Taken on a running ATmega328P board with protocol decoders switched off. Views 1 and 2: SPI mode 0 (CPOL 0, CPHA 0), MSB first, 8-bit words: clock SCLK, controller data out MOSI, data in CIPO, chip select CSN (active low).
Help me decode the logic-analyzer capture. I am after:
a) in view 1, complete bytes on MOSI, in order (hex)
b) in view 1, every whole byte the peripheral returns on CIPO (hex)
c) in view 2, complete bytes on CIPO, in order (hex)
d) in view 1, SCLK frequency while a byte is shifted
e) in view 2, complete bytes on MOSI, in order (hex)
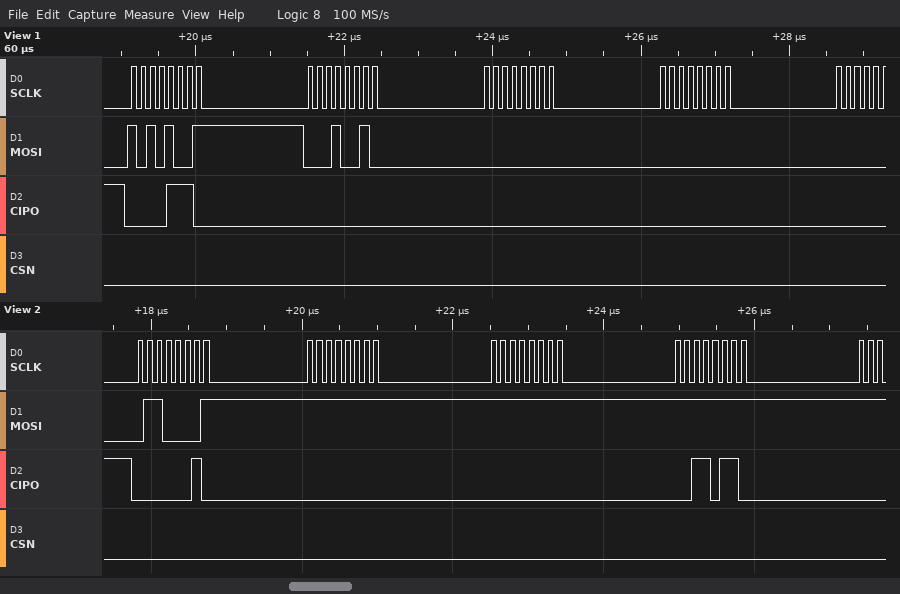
0xA9 0x12 0x00 0x00
0x0E 0x00 0x00 0x00
02 00 00 36
8 MHz
61 FF FF FF
